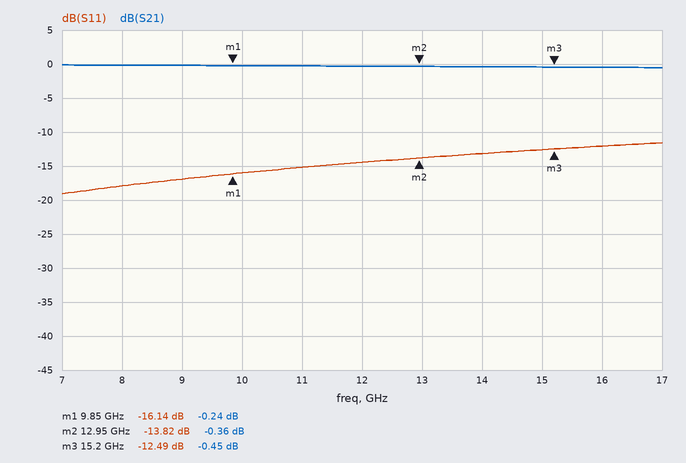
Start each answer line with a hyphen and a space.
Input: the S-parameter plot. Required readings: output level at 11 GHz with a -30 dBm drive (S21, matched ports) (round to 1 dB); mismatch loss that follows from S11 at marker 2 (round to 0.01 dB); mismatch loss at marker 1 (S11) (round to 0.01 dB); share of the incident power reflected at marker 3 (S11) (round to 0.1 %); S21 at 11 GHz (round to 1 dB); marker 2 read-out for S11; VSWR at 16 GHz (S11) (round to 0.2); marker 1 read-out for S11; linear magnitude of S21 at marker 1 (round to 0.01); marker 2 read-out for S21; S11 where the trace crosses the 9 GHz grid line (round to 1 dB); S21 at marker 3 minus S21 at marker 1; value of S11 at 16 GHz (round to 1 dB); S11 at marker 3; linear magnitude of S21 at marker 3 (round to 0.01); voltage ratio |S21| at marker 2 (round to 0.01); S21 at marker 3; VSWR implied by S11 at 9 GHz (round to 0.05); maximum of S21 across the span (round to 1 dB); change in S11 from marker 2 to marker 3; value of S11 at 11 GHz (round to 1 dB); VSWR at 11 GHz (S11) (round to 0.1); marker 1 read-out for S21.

- -30 dBm
- 0.18 dB
- 0.11 dB
- 5.6 %
- 0 dB
- -13.82 dB
- 1.6
- -16.14 dB
- 0.97
- -0.36 dB
- -17 dB
- -0.21 dB
- -12 dB
- -12.49 dB
- 0.95
- 0.96
- -0.45 dB
- 1.35
- 0 dB
- 1.33 dB
- -15 dB
- 1.4
- -0.24 dB
